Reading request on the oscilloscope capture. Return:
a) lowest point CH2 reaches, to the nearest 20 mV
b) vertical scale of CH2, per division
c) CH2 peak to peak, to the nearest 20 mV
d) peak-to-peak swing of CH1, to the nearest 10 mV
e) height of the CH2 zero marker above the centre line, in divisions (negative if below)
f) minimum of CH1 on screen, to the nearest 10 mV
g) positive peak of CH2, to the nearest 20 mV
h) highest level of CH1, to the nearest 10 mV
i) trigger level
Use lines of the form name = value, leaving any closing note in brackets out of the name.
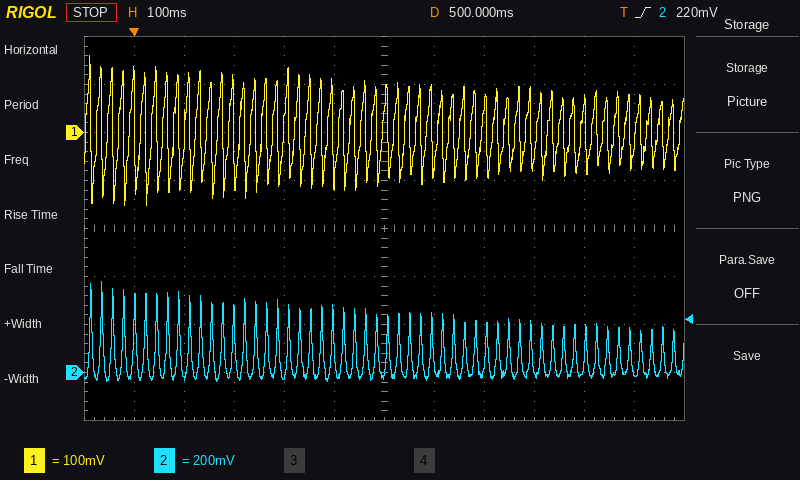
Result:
lowest point CH2 reaches, to the nearest 20 mV = -40 mV
vertical scale of CH2, per division = 200 mV
CH2 peak to peak, to the nearest 20 mV = 420 mV
peak-to-peak swing of CH1, to the nearest 10 mV = 310 mV
height of the CH2 zero marker above the centre line, in divisions = -3.0 div
minimum of CH1 on screen, to the nearest 10 mV = -150 mV
positive peak of CH2, to the nearest 20 mV = 380 mV
highest level of CH1, to the nearest 10 mV = 160 mV
trigger level = 220 mV
